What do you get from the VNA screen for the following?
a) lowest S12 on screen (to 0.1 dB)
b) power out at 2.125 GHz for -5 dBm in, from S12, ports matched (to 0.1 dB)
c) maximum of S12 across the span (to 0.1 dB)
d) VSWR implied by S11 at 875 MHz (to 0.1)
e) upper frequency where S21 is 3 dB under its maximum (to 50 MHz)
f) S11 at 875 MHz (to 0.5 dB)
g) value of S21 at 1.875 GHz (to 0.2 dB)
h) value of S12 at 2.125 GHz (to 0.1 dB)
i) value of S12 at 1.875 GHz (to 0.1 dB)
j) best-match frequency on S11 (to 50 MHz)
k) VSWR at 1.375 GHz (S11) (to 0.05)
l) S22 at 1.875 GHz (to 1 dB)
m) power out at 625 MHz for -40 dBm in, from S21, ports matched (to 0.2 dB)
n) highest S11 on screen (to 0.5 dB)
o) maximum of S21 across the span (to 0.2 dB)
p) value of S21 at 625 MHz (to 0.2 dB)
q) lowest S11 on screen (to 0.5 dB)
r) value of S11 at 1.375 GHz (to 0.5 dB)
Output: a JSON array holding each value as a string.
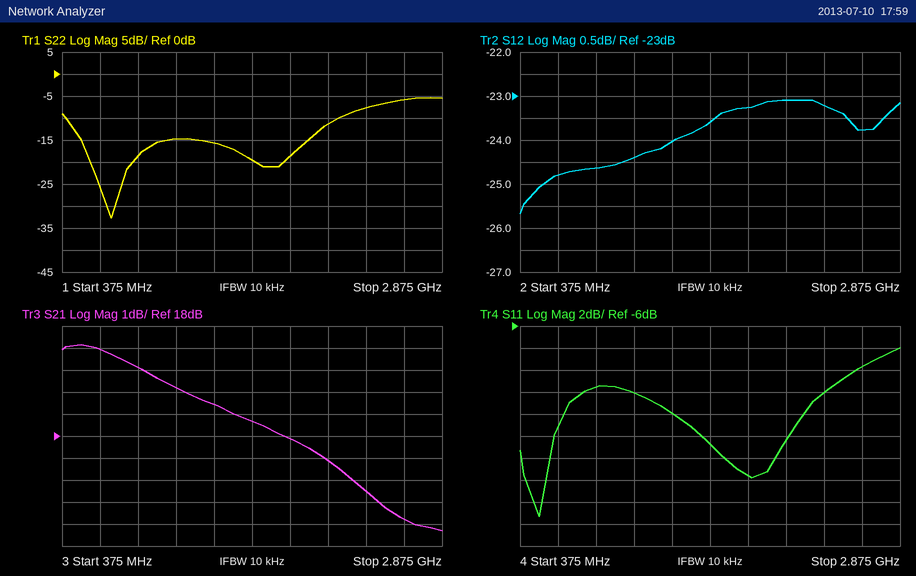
["-25.7 dB", "-28.1 dBm", "-23.1 dB", "1.7", "1.45 GHz", "-11.5 dB", "17.8 dB", "-23.1 dB", "-23.3 dB", "500 MHz", "1.50", "-19 dB", "-18.0 dBm", "-8.0 dB", "22.2 dB", "22.0 dB", "-23.5 dB", "-14.0 dB"]
